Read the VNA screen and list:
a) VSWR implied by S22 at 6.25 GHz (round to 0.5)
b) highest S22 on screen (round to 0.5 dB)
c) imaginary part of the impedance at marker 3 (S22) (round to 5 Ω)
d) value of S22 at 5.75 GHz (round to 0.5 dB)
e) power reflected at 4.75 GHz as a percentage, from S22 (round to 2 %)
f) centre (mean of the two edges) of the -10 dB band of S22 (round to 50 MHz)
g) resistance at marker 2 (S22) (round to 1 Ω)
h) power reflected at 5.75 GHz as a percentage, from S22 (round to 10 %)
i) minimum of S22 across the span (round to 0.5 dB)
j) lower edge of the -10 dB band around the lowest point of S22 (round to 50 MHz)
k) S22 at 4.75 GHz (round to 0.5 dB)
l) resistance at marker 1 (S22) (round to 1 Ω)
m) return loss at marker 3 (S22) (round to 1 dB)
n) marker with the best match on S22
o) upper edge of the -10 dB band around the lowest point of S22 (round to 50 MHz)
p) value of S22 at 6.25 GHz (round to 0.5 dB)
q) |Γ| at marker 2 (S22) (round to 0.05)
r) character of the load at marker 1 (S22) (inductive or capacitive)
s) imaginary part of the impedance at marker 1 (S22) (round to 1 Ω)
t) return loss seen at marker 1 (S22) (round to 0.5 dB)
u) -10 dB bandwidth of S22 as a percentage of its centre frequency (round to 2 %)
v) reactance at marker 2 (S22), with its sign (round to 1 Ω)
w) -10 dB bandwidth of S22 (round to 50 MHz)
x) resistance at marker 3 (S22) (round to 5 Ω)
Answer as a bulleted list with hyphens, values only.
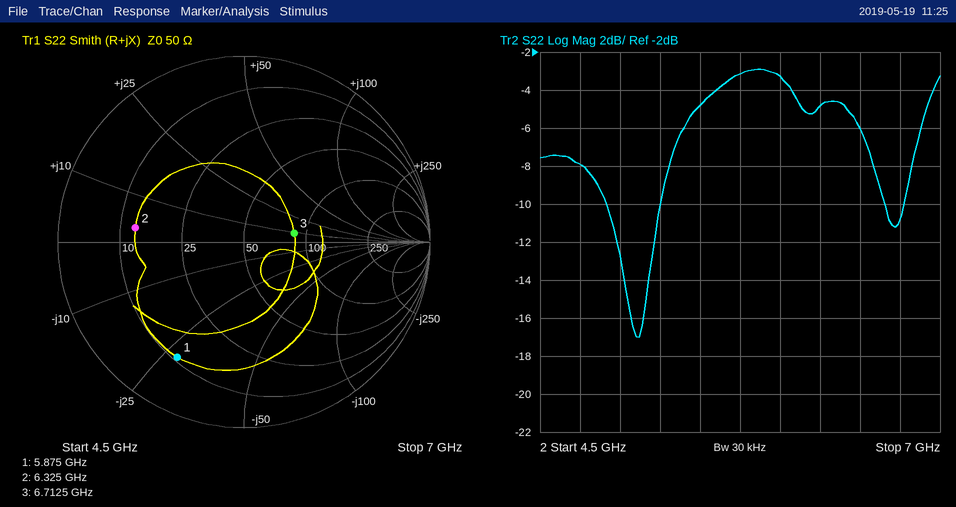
- 3.5
- -3.0 dB
- +10 Ω
- -3.0 dB
- 16 %
- 5.10 GHz
- 13 Ω
- 50 %
- -17.0 dB
- 4.90 GHz
- -8.0 dB
- 11 Ω
- 11 dB
- marker 3
- 5.25 GHz
- -5.0 dB
- 0.60
- capacitive
- -28 Ω
- 3.0 dB
- 6 %
- +3 Ω
- 350 MHz
- 85 Ω
